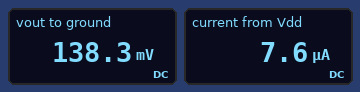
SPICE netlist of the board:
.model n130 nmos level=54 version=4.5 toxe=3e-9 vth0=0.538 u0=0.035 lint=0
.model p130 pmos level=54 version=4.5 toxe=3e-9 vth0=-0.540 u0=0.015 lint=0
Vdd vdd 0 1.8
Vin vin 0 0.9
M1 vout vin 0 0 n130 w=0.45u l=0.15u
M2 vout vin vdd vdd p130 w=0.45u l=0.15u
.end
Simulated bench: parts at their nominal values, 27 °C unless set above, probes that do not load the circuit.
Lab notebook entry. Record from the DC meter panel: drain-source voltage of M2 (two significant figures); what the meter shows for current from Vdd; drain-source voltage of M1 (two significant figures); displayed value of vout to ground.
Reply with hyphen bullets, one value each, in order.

- -1.7 V
- 7.6 µA
- 140 mV
- 138.3 mV
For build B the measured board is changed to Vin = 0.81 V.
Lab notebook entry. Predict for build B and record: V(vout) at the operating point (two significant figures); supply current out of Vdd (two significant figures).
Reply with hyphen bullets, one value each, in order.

- 1.7 V
- 6.1 µA
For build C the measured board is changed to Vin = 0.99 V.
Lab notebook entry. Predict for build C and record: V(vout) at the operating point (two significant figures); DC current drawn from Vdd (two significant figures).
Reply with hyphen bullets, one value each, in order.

- 17 mV
- 2.5 µA
